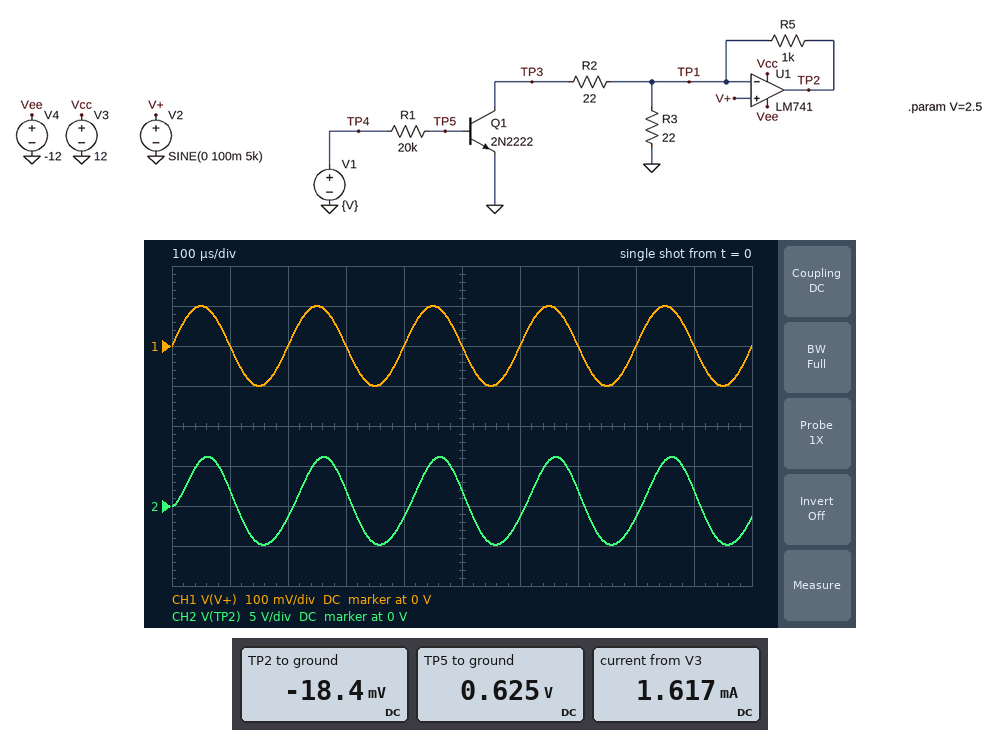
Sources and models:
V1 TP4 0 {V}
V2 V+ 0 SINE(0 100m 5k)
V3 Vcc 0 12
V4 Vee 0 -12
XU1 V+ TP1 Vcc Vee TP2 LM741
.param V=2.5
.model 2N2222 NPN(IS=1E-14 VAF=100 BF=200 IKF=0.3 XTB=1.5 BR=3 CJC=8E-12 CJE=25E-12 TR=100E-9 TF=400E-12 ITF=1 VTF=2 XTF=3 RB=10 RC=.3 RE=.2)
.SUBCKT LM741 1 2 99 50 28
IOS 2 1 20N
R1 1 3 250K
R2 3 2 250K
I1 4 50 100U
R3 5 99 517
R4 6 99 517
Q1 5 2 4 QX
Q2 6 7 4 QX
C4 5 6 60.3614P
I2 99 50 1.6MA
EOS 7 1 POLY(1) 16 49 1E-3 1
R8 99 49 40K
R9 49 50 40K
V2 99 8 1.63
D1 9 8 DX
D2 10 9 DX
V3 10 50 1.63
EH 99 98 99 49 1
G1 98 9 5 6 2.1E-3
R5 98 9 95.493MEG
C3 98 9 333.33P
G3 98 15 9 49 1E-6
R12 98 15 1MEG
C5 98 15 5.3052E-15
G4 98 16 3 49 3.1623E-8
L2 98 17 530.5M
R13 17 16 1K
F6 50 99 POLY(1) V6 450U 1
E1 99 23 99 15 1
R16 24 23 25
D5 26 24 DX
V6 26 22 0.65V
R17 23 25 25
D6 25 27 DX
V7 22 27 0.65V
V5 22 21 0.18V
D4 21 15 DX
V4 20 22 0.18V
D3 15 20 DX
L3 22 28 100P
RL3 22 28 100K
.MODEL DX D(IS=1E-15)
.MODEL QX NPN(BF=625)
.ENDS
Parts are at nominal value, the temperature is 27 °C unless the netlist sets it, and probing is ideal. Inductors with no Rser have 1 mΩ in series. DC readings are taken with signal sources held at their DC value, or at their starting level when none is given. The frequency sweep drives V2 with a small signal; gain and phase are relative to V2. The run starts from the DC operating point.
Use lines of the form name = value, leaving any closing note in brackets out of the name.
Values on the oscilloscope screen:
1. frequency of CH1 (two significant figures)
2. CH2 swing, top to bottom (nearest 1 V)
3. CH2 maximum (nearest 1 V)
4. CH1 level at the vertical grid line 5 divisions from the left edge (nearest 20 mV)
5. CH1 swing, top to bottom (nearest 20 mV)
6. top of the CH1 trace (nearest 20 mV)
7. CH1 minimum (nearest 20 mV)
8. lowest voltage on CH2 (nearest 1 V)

frequency of CH1 = 5.0 kHz
CH2 swing, top to bottom = 11 V
CH2 maximum = 6 V
CH1 level at the vertical grid line 5 divisions from the left edge = 0 V
CH1 swing, top to bottom = 200 mV
top of the CH1 trace = 100 mV
CH1 minimum = -100 mV
lowest voltage on CH2 = -5 V
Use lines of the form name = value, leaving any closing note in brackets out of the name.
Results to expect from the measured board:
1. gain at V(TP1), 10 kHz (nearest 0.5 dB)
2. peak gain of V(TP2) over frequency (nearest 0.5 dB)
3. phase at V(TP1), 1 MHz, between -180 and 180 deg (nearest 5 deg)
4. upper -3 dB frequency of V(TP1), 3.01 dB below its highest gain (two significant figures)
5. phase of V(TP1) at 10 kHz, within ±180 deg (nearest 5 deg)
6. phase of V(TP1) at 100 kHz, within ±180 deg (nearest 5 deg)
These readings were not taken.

gain at V(TP1), 10 kHz = -1.5 dB
peak gain of V(TP2) over frequency = 35.0 dB
phase at V(TP1), 1 MHz, between -180 and 180 deg = -110 deg
upper -3 dB frequency of V(TP1), 3.01 dB below its highest gain = 15 kHz
phase of V(TP1) at 10 kHz, within ±180 deg = -35 deg
phase of V(TP1) at 100 kHz, within ±180 deg = -85 deg
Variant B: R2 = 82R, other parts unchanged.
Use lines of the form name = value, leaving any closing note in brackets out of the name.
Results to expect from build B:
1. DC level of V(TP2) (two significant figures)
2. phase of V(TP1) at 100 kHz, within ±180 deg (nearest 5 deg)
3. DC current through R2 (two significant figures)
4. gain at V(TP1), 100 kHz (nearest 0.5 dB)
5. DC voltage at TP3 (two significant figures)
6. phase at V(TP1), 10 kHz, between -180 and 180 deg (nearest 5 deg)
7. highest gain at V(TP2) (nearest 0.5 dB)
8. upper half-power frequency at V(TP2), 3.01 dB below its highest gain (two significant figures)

DC level of V(TP2) = 5.2 mV
phase of V(TP1) at 100 kHz, within ±180 deg = -85 deg
DC current through R2 = 41 µA
gain at V(TP1), 100 kHz = -16.0 dB
DC voltage at TP3 = 4.4 mV
phase at V(TP1), 10 kHz, between -180 and 180 deg = -30 deg
highest gain at V(TP2) = 34.5 dB
upper half-power frequency at V(TP2), 3.01 dB below its highest gain = 16 kHz
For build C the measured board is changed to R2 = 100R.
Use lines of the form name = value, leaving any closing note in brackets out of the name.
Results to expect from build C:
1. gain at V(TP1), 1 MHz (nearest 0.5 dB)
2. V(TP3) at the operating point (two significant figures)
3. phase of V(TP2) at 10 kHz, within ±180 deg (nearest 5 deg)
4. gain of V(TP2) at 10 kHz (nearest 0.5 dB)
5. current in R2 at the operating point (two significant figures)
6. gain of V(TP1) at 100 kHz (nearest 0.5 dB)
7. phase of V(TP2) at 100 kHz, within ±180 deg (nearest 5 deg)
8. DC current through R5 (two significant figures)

gain at V(TP1), 1 MHz = -36.5 dB
V(TP3) at the operating point = 4.7 mV
phase of V(TP2) at 10 kHz, within ±180 deg = -30 deg
gain of V(TP2) at 10 kHz = 33.0 dB
current in R2 at the operating point = 37 µA
gain of V(TP1) at 100 kHz = -16.0 dB
phase of V(TP2) at 100 kHz, within ±180 deg = -85 deg
DC current through R5 = 8.4 µA
